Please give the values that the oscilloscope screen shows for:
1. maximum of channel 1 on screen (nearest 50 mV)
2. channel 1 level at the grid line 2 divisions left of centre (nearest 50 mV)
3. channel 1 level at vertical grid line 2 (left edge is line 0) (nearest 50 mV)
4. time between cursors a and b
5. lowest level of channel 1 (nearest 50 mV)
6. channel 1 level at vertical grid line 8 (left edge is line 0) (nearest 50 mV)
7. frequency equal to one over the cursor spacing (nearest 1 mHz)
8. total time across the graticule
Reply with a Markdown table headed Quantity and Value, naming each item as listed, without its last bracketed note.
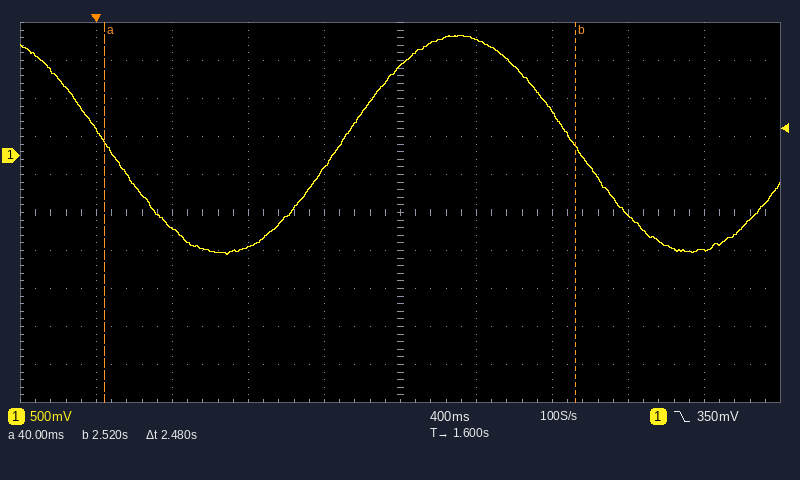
| Quantity | Value |
|---|---|
| maximum of channel 1 on screen | 1.60 V |
| channel 1 level at the grid line 2 divisions left of centre | -1.20 V |
| channel 1 level at vertical grid line 2 (left edge is line 0) | -950 mV |
| time between cursors a and b | 2.48 s |
| lowest level of channel 1 | -1.30 V |
| channel 1 level at vertical grid line 8 (left edge is line 0) | -800 mV |
| frequency equal to one over the cursor spacing | 403 mHz |
| total time across the graticule | 4 s |
